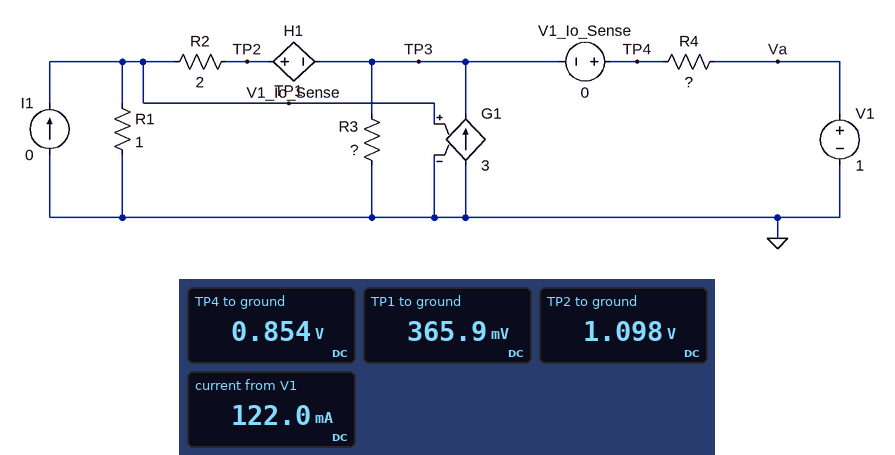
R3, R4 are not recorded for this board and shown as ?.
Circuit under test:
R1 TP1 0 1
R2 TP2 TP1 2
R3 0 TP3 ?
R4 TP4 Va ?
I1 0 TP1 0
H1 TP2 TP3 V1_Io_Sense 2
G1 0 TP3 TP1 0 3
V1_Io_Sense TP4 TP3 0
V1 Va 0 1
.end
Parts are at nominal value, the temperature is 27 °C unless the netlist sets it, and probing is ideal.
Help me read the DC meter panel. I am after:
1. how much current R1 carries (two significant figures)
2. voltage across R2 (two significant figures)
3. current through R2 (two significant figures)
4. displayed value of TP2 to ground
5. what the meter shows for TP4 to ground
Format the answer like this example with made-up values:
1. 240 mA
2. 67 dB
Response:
1. 370 mA
2. 730 mV
3. 370 mA
4. 1.098 V
5. 0.854 V
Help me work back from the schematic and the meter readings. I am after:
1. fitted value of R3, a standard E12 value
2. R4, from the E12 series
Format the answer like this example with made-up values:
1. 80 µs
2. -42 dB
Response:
1. 1 Ω
2. 1.2 Ω
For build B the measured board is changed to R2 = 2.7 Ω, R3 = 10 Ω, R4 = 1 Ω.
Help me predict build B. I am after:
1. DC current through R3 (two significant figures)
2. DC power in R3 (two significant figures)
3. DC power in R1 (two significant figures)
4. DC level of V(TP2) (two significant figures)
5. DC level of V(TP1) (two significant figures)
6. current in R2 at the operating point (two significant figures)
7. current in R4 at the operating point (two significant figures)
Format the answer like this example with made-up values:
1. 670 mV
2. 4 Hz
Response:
1. 130 mA
2. 160 mW
3. 39 mW
4. 730 mV
5. 200 mV
6. 200 mA
7. 270 mA
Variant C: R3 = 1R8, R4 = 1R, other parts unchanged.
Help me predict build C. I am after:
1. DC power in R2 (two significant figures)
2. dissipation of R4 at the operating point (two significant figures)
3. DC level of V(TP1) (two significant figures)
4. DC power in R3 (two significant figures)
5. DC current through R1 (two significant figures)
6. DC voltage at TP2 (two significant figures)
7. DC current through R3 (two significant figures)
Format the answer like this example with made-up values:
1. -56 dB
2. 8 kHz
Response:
1. 200 mW
2. 2.5 mW
3. 320 mV
4. 610 mW
5. 320 mA
6. 950 mV
7. 580 mA
